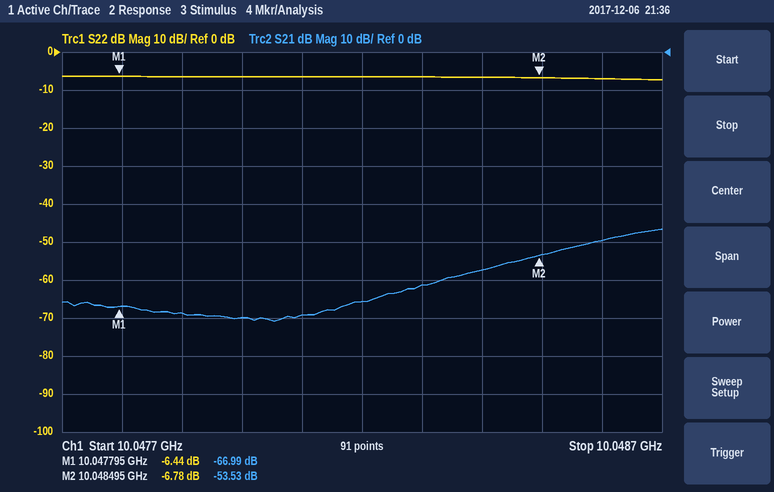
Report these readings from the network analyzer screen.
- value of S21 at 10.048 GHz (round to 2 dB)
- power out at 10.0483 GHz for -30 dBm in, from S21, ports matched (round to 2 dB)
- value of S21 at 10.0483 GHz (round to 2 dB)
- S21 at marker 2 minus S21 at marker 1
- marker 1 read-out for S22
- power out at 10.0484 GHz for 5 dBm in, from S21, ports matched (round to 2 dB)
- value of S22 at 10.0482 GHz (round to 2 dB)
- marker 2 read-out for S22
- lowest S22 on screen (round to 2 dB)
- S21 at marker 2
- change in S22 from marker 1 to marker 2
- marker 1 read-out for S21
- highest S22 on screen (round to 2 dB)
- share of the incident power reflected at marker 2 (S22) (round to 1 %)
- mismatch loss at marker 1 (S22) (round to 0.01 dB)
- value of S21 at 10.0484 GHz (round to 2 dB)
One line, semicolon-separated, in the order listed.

-70 dB; -92 dBm; -62 dB; 13.46 dB; -6.44 dB; -52 dBm; -6 dB; -6.78 dB; -8 dB; -53.53 dB; -0.34 dB; -66.99 dB; -6 dB; 21 %; 1.12 dB; -58 dB
